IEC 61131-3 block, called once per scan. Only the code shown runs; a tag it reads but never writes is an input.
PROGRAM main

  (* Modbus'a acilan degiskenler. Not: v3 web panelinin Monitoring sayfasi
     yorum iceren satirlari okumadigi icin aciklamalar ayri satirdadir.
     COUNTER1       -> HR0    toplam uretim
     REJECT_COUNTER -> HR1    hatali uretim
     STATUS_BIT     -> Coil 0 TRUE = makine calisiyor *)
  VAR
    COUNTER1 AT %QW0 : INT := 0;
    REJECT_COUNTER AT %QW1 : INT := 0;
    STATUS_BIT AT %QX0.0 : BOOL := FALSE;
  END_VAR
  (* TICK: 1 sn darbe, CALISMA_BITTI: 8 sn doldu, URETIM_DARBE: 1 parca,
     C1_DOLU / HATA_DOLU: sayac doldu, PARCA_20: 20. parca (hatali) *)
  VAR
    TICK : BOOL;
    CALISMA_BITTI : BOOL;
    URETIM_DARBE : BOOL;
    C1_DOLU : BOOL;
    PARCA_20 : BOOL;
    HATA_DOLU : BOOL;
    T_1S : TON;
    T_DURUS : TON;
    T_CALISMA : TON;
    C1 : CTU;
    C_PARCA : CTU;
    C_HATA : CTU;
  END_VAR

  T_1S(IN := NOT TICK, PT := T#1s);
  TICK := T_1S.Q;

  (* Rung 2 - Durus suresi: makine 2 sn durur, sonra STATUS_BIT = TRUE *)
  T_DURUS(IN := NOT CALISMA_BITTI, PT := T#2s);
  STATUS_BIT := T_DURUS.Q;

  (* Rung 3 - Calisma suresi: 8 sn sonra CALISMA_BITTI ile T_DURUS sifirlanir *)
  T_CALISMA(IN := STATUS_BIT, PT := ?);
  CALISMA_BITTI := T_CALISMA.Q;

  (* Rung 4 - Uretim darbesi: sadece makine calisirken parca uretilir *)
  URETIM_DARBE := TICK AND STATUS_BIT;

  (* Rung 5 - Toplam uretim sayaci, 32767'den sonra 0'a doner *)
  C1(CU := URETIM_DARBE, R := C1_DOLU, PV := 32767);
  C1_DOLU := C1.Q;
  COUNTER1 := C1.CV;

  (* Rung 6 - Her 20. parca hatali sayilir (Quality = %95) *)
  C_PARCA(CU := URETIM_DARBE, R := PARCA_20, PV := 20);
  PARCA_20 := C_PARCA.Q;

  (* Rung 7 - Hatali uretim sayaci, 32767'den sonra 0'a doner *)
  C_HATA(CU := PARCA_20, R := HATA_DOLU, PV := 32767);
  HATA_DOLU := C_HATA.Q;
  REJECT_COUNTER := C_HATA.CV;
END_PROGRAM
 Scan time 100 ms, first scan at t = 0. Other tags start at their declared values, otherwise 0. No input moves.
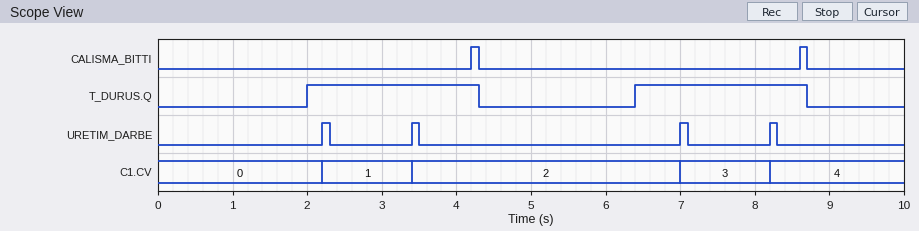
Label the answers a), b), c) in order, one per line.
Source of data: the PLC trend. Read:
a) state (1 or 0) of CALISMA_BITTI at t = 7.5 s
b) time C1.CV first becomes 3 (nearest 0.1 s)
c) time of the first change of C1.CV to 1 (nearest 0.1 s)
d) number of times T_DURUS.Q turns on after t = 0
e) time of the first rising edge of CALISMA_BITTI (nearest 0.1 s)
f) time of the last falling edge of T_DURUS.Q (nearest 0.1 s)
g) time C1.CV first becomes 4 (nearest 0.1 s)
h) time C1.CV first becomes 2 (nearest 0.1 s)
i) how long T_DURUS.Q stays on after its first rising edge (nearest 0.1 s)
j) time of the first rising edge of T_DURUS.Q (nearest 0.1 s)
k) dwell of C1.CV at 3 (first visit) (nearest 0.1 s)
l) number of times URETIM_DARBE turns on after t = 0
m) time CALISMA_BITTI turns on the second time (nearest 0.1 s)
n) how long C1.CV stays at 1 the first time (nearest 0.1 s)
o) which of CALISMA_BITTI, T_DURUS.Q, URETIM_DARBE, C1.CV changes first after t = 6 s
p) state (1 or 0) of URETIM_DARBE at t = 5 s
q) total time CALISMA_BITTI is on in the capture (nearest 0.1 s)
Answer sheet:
a) 0
b) 7.0 s
c) 2.2 s
d) 2
e) 4.2 s
f) 8.7 s
g) 8.2 s
h) 3.4 s
i) 2.3 s
j) 2.0 s
k) 1.2 s
l) 4
m) 8.6 s
n) 1.2 s
o) T_DURUS.Q
p) 0
q) 0.2 s
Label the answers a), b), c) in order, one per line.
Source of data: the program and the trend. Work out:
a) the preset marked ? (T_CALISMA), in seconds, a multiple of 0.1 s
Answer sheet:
a) 2.2 s
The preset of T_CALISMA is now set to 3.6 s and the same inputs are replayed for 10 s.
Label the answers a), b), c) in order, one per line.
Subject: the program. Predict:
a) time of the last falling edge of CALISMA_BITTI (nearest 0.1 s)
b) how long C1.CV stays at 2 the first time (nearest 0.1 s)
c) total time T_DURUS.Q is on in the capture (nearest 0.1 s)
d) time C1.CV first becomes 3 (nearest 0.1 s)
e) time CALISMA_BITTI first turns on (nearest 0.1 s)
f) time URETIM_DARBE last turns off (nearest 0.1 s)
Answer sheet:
a) 5.7 s
b) 1.2 s
c) 5.9 s
d) 4.6 s
e) 5.6 s
f) 9.5 s
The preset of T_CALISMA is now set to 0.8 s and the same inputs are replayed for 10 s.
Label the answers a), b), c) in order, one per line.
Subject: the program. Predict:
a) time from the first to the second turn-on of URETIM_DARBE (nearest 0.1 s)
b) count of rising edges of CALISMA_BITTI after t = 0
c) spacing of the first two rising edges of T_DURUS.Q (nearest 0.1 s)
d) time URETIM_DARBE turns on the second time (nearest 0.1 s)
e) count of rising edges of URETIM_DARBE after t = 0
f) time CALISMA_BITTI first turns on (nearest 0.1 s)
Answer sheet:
a) 3.6 s
b) 3
c) 3.0 s
d) 5.8 s
e) 3
f) 2.8 s
